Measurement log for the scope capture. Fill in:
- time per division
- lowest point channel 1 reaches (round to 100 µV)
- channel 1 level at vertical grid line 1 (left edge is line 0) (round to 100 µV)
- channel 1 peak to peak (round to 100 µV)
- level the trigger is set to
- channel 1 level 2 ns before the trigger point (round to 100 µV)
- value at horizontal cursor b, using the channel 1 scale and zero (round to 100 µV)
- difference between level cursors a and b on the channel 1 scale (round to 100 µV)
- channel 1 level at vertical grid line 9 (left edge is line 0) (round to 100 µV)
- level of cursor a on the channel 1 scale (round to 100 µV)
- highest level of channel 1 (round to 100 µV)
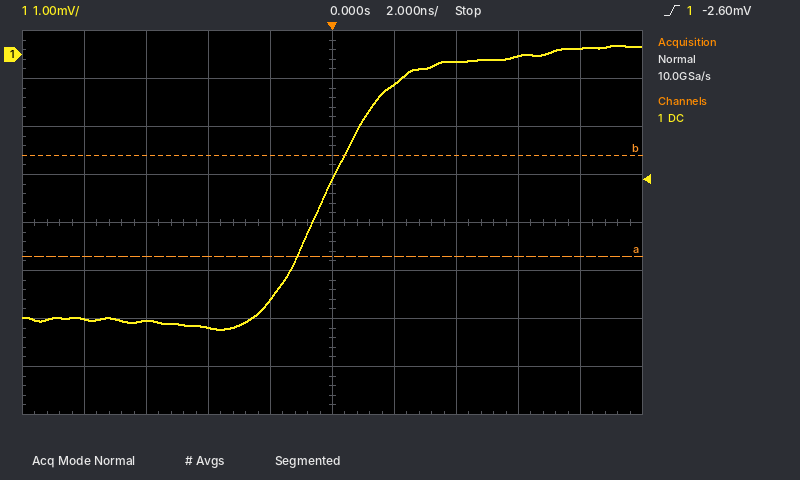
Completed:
2 ns
-5.7 mV
-5.5 mV
5.9 mV
-2.60 mV
-5.1 mV
-2.1 mV
2.1 mV
100 µV
-4.2 mV
200 µV
